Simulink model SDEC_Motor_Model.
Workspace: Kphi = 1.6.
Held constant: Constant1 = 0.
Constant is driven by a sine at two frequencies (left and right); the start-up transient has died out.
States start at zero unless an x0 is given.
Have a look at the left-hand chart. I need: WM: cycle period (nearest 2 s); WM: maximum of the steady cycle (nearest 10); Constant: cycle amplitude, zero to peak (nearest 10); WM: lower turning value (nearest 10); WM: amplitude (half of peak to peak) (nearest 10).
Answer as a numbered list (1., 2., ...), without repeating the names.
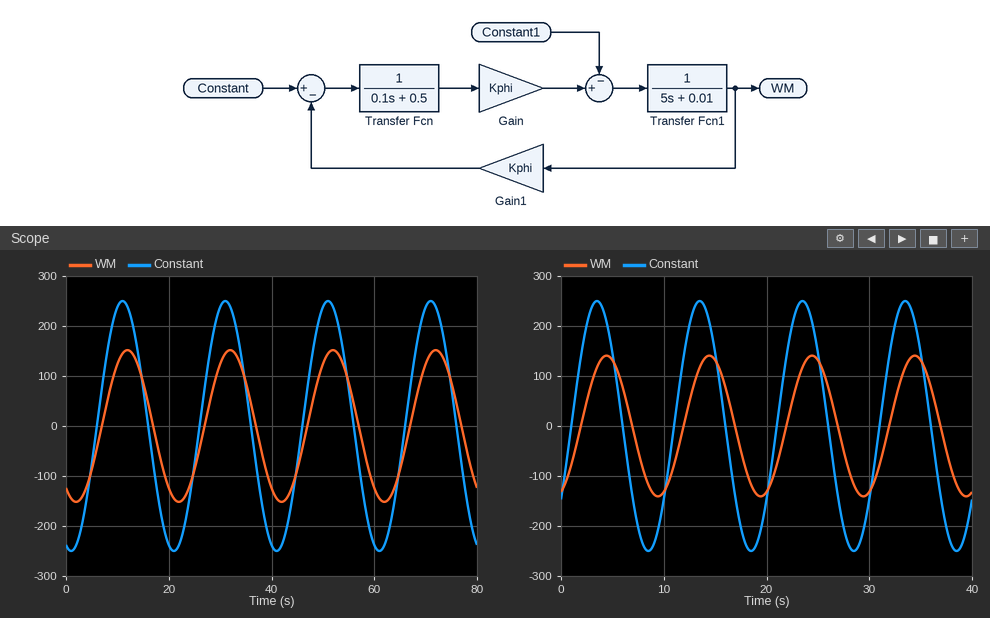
1. 20 s
2. 150
3. 250
4. -150
5. 150
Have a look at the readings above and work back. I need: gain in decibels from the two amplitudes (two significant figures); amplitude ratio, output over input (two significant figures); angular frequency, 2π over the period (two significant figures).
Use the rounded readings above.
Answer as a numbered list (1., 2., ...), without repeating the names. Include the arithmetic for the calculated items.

1. 20 log10(150 / 250) = -4.4 dB
2. 150 / 250 = 0.60
3. 2π / 20 = 0.31 rad/s
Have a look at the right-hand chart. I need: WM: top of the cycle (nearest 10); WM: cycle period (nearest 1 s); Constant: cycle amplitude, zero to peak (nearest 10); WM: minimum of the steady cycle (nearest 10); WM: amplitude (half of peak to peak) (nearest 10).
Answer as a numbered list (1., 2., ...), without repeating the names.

1. 140
2. 10 s
3. 250
4. -140
5. 140
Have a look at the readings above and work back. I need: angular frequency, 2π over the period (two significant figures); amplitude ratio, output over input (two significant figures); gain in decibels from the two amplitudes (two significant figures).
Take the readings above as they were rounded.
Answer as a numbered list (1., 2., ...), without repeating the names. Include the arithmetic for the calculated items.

1. 2π / 10 = 0.63 rad/s
2. 140 / 250 = 0.56
3. 20 log10(140 / 250) = -5.0 dB
